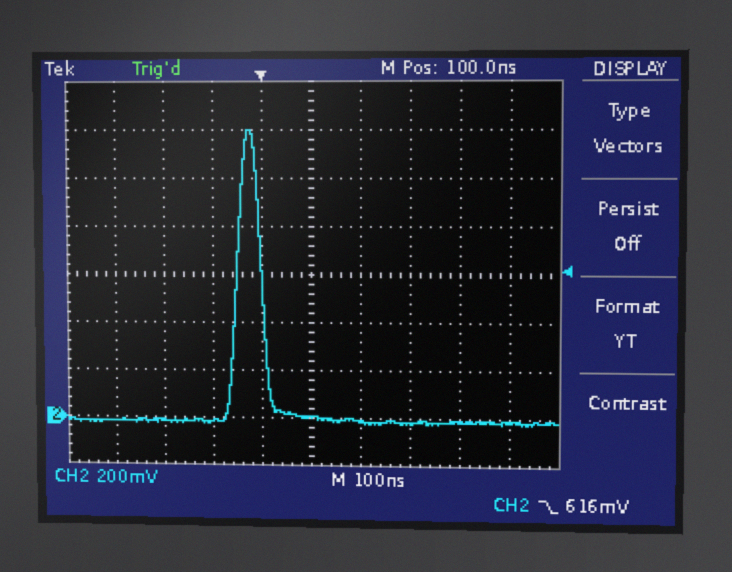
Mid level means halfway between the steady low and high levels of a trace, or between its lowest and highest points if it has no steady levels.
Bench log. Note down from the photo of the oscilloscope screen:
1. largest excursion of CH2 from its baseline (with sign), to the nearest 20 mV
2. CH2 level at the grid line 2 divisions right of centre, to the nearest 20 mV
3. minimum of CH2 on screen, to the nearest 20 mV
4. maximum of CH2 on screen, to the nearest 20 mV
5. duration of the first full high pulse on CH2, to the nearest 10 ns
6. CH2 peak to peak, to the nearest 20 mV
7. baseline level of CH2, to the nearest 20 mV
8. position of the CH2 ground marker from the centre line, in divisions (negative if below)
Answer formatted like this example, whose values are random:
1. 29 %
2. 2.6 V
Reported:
1. +1.22 V
2. -20 mV
3. -20 mV
4. 1.20 V
5. 50 ns
6. 1.22 V
7. -20 mV
8. -3.0 div
